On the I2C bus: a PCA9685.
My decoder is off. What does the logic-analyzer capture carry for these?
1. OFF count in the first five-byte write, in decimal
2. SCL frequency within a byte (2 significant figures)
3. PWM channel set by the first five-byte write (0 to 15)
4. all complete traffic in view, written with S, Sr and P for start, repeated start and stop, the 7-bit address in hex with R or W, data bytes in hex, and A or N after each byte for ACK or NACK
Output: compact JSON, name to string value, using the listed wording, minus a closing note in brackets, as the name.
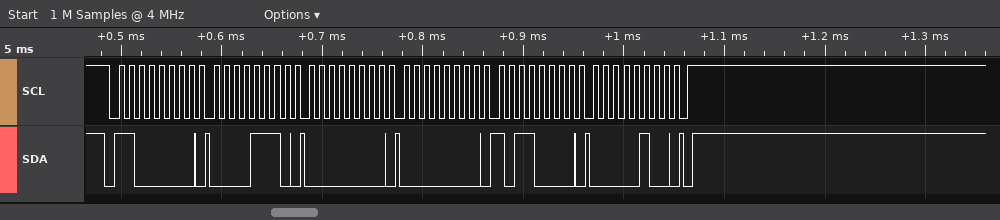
{"OFF count in the first five-byte write, in decimal": "1200", "SCL frequency within a byte": "100 kHz", "PWM channel set by the first five-byte write": "2", "all complete traffic in view, written with S, Sr and P for start, repeated start and stop, the 7-bit address in hex with R or W, data bytes in hex, and A or N after each byte for ACK or NACK": "S 60W A 0E A 00 A 00 A B0 A 04 A P"}
